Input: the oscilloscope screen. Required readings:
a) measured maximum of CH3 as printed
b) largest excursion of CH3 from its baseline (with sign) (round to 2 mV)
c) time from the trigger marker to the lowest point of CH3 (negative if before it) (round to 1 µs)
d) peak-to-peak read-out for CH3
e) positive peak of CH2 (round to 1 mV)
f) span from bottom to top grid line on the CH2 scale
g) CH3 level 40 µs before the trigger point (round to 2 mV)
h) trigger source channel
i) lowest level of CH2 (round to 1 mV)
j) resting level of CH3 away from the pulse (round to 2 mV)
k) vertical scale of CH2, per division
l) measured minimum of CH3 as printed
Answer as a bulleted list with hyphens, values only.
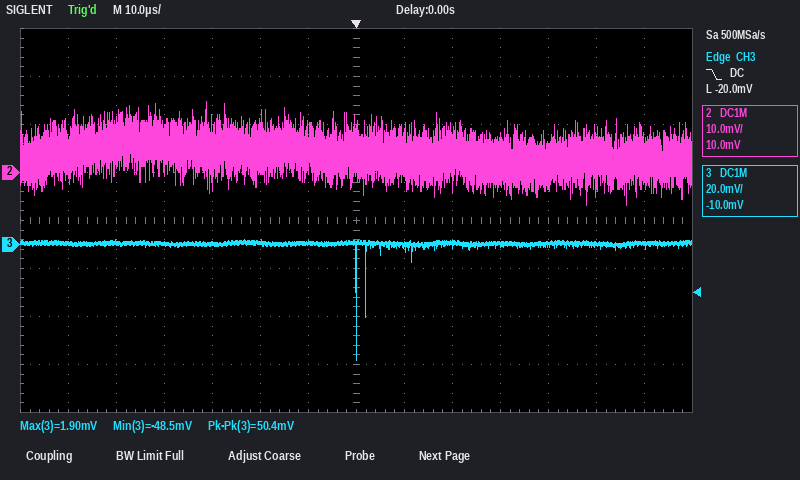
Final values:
- 1.90 mV
- -48 mV
- 0 µs
- 50.4 mV
- 15 mV
- 80 mV
- 0 mV
- CH3
- -7 mV
- 0 mV
- 10 mV
- -48.5 mV
